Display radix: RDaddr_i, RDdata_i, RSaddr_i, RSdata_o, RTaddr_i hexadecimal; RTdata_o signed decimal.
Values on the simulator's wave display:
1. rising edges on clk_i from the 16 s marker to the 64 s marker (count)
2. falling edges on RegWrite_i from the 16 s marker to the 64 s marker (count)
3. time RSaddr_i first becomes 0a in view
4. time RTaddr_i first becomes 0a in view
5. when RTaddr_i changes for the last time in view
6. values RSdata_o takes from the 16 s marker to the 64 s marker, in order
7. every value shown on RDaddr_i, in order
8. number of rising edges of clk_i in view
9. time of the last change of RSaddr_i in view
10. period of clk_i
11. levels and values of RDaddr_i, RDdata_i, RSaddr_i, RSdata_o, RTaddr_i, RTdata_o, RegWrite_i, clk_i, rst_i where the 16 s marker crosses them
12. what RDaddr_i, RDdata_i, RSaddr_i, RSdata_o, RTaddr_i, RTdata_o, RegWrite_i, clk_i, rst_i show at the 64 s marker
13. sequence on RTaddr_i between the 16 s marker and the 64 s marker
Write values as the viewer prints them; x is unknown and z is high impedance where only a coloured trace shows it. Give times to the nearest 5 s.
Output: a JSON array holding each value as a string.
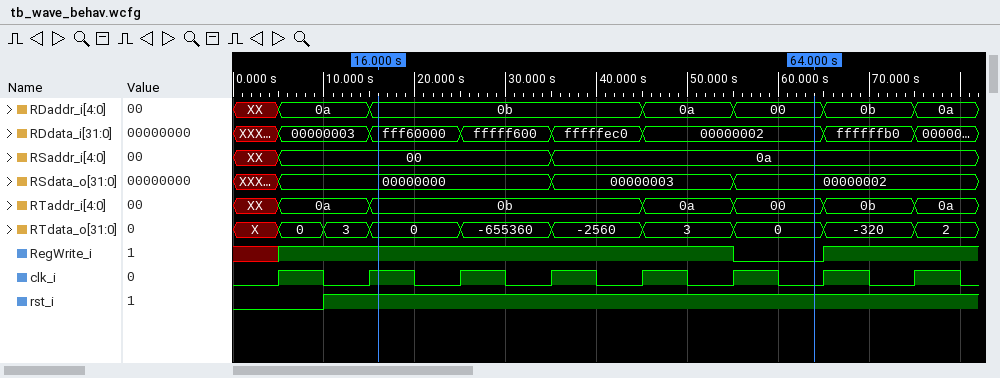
["4", "1", "35 s", "5 s", "75 s", "00000000, 00000003, 00000002", "XX, 0a, 0b, 0a, 00, 0b, 0a", "8", "35 s", "10 s", "RDaddr_i=0b, RDdata_i=fff60000, RSaddr_i=00, RSdata_o=00000000, RTaddr_i=0b, RTdata_o=0, RegWrite_i=1, clk_i=1, rst_i=1", "RDaddr_i=00, RDdata_i=00000002, RSaddr_i=0a, RSdata_o=00000002, RTaddr_i=00, RTdata_o=0, RegWrite_i=0, clk_i=0, rst_i=1", "0b, 0a, 00"]
